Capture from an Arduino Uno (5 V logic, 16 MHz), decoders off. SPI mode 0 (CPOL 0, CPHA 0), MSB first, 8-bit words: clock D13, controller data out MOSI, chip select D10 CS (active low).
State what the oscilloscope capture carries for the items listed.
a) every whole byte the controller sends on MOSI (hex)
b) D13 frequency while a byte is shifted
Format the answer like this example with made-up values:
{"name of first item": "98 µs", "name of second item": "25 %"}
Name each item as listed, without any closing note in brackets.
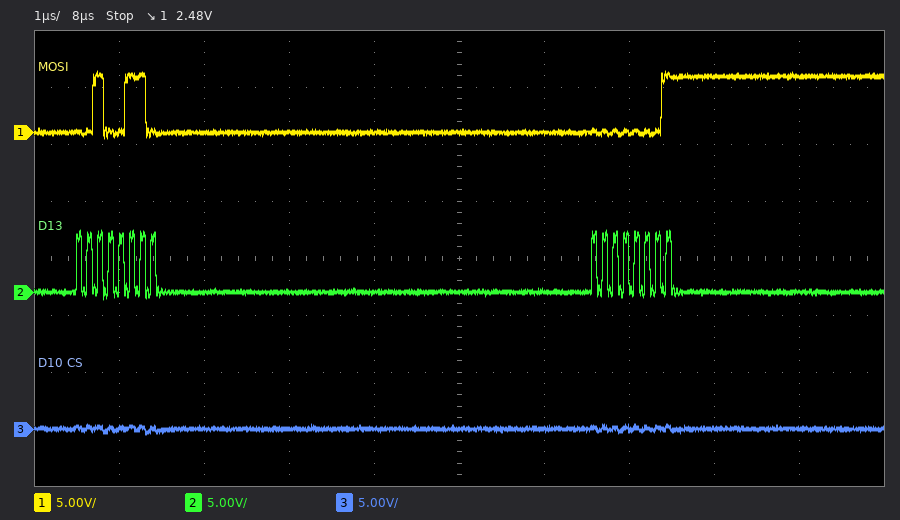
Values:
{"every whole byte the controller sends on MOSI": "0x26 0x01", "D13 frequency while a byte is shifted": "8 MHz"}
